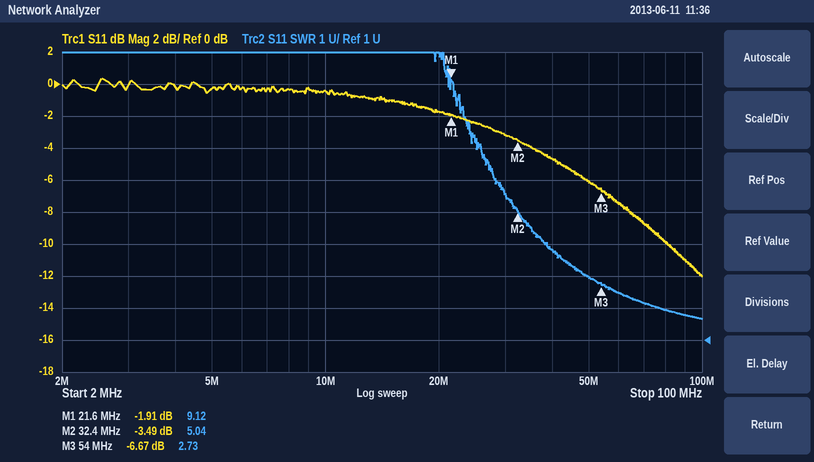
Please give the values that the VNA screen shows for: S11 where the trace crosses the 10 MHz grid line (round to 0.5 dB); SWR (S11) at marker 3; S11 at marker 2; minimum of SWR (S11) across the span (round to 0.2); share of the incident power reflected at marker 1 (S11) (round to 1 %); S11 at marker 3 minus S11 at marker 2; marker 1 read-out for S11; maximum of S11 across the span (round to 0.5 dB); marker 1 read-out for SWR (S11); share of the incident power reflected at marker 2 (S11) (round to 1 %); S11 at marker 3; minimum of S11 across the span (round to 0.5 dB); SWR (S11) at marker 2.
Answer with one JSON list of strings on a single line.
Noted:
["-0.5 dB", "2.73", "-3.49 dB", "1.6", "64 %", "-3.18 dB", "-1.91 dB", "0.5 dB", "9.12", "45 %", "-6.67 dB", "-12.0 dB", "5.04"]
